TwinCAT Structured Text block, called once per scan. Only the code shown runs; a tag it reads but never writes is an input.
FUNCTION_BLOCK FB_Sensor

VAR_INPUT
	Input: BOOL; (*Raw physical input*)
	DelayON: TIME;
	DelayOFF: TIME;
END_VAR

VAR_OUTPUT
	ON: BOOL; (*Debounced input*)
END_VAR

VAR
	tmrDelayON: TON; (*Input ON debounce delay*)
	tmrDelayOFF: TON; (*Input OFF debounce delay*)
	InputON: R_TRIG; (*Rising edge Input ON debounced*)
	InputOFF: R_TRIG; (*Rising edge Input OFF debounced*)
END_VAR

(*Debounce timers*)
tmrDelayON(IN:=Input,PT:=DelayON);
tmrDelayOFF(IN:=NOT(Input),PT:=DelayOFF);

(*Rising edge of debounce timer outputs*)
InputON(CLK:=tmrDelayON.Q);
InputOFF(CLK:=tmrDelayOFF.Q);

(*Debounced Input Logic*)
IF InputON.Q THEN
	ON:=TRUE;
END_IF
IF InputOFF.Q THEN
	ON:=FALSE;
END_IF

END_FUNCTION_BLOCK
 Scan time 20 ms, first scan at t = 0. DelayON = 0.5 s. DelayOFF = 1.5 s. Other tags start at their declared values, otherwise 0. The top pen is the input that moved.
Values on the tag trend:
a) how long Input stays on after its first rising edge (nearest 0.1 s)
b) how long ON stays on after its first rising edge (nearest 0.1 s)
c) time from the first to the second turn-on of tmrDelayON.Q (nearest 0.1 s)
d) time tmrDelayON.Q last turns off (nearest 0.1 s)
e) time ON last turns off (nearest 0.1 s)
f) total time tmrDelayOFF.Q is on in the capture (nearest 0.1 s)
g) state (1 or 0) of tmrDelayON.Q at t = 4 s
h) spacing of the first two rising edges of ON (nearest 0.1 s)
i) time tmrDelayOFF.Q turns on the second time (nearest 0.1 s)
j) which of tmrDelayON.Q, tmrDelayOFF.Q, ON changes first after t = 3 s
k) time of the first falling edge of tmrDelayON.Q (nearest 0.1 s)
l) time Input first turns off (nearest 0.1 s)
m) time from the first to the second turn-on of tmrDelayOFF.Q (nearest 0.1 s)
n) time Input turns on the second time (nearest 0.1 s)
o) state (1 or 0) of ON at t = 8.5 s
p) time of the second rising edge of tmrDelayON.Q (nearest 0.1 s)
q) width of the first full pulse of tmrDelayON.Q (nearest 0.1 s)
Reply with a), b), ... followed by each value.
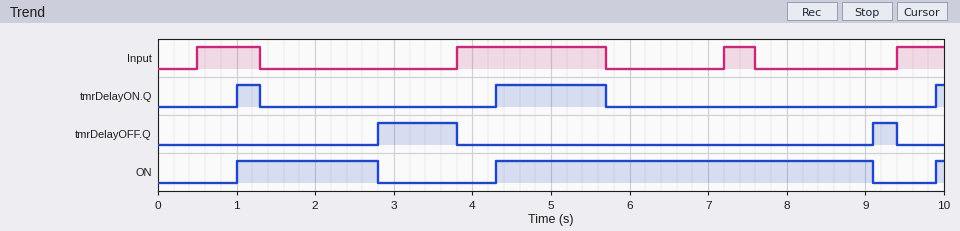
a) 0.8 s
b) 1.8 s
c) 3.3 s
d) 5.7 s
e) 9.1 s
f) 1.3 s
g) 0
h) 3.3 s
i) 9.1 s
j) tmrDelayOFF.Q
k) 1.3 s
l) 1.3 s
m) 6.3 s
n) 3.8 s
o) 1
p) 4.3 s
q) 0.3 s
